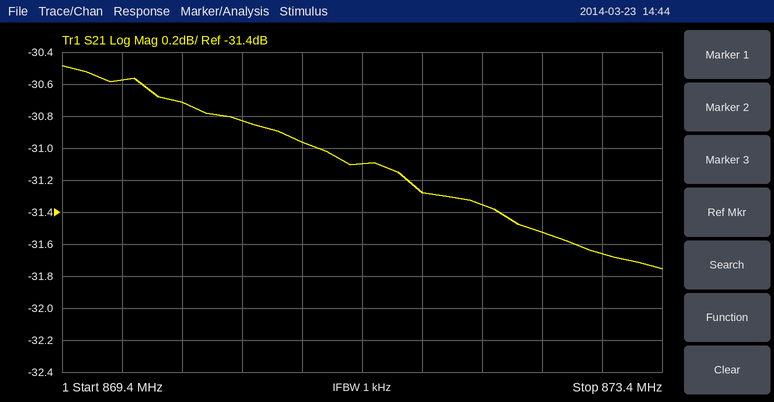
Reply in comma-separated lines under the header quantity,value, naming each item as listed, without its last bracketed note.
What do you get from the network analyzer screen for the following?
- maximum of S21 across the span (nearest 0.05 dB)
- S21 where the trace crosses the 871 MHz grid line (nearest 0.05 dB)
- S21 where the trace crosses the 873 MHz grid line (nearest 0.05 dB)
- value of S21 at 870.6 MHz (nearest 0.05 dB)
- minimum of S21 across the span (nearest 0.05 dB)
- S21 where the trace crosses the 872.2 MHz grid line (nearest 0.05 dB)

quantity,value
maximum of S21 across the span,-30.50 dB
S21 where the trace crosses the 871 MHz grid line,-30.95 dB
S21 where the trace crosses the 873 MHz grid line,-31.65 dB
value of S21 at 870.6 MHz,-30.85 dB
minimum of S21 across the span,-31.75 dB
S21 where the trace crosses the 872.2 MHz grid line,-31.35 dB
